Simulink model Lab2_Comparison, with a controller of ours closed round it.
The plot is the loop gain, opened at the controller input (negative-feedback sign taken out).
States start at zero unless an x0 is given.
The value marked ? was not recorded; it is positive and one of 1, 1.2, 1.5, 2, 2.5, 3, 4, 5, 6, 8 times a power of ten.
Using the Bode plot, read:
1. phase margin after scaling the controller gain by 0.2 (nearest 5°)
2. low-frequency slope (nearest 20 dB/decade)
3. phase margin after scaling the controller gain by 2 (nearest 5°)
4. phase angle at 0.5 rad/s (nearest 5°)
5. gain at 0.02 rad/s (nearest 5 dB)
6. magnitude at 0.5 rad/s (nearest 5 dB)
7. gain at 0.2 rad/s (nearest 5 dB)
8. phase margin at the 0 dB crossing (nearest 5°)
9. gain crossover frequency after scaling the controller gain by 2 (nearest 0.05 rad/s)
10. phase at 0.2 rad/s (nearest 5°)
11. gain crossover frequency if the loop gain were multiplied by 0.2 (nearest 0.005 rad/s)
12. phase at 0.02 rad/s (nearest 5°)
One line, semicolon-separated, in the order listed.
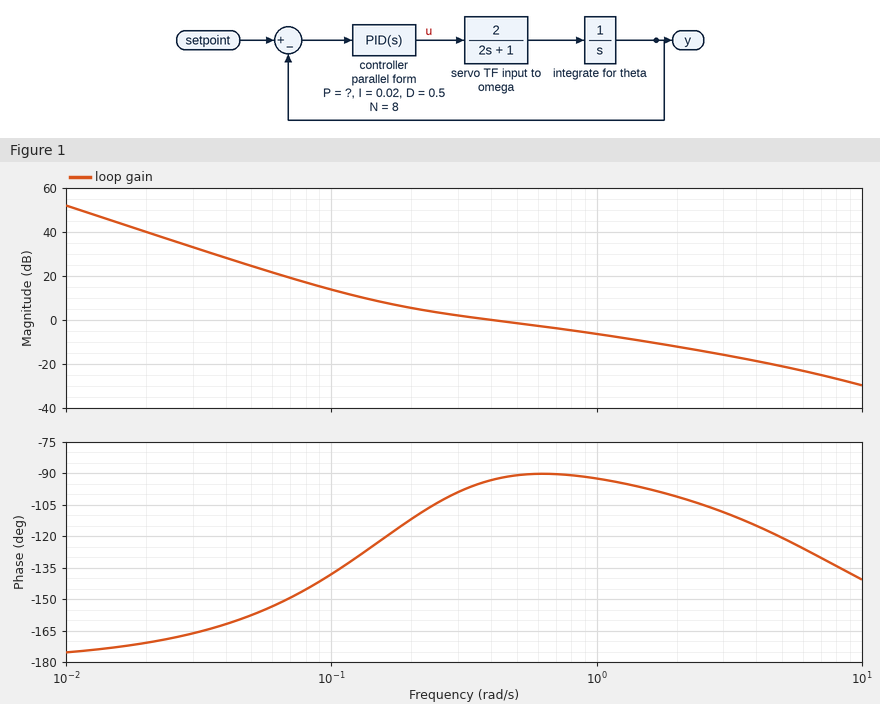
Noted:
40°; -40 dB/decade; 90°; -90°; 40 dB; 0 dB; 5 dB; 85°; 0.95 rad/s; -110°; 0.100 rad/s; -170°
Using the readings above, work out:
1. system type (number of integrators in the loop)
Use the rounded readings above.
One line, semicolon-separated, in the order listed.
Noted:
2
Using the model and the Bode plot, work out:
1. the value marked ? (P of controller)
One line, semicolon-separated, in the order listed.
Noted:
0.2
